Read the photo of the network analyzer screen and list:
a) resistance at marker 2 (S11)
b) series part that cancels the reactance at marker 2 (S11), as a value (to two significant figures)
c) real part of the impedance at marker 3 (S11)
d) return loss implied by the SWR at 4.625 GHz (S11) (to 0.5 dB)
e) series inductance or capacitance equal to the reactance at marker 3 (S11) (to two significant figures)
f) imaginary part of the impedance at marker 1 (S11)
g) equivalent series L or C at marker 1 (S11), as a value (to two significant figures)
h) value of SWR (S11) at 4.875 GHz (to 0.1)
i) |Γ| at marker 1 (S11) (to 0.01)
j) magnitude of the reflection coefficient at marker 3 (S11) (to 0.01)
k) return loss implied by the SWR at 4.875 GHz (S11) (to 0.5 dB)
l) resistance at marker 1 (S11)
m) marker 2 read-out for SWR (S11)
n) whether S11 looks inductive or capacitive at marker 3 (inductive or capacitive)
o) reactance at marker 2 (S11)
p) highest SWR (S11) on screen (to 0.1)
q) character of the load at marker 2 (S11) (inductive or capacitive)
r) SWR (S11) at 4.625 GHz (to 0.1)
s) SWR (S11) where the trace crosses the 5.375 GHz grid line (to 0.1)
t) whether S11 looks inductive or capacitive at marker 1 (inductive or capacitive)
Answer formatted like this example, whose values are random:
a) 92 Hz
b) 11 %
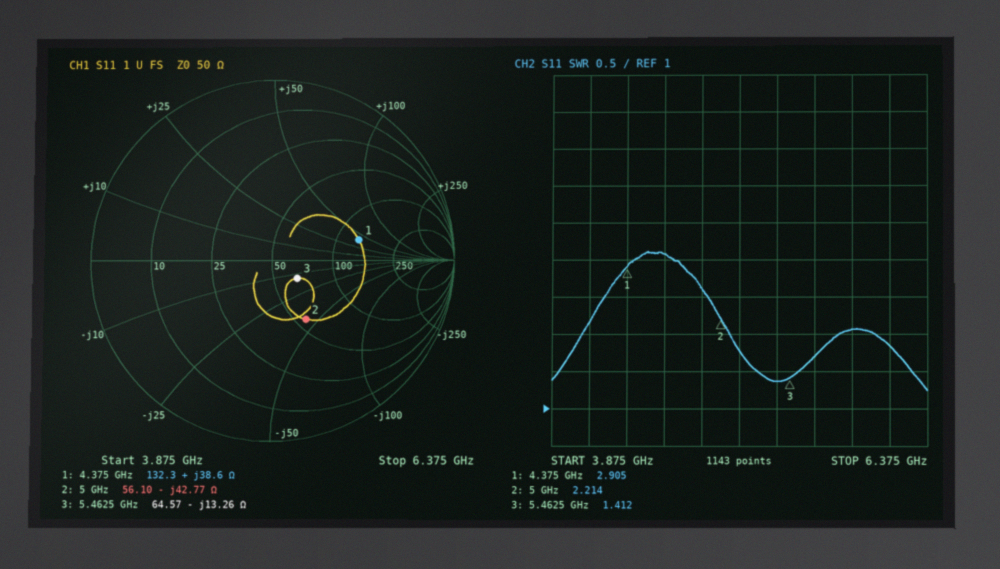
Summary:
a) 56.10 Ω
b) 1.4 nH
c) 64.57 Ω
d) 6.0 dB
e) 2.2 pF
f) +38.6 Ω
g) 1.4 nH
h) 2.6
i) 0.49
j) 0.17
k) 7.0 dB
l) 132.3 Ω
m) 2.214
n) capacitive
o) -42.77 Ω
p) 3.1
q) capacitive
r) 3.1
s) 1.4
t) inductive
